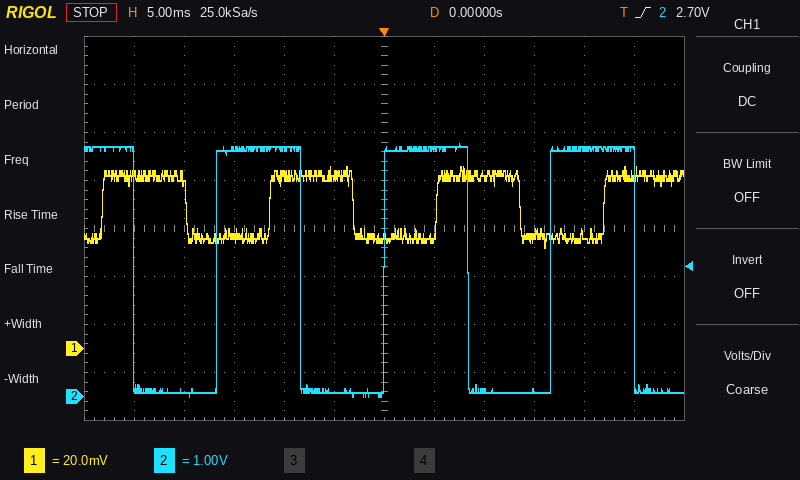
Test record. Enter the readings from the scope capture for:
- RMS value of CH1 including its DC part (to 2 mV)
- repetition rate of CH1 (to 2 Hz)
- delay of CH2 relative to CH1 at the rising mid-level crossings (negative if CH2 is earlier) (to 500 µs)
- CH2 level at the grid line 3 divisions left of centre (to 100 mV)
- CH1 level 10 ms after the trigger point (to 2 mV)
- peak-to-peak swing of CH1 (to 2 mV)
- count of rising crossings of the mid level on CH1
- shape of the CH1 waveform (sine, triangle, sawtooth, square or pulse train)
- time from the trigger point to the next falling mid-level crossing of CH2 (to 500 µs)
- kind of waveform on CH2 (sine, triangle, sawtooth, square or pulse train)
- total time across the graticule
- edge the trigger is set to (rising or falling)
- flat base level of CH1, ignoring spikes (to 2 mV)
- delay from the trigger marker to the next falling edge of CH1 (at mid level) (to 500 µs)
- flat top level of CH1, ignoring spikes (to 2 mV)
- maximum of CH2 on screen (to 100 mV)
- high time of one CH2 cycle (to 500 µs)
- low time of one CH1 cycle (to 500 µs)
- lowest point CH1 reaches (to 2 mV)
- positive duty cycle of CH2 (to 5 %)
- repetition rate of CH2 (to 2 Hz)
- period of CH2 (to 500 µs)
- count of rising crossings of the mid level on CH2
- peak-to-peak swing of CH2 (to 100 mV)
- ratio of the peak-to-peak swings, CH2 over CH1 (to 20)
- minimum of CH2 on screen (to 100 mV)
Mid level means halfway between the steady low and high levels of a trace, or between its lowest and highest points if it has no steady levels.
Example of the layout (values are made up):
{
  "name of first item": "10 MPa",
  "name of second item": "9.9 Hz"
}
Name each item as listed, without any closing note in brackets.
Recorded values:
{
  "RMS value of CH1 including its DC part": "60 mV",
  "repetition rate of CH1": "60 Hz",
  "delay of CH2 relative to CH1 at the rising mid-level crossings (negative if CH2 is earlier)": "-5.5 ms",
  "CH2 level at the grid line 3 divisions left of centre": "5.2 V",
  "CH1 level 10 ms after the trigger point": "72 mV",
  "peak-to-peak swing of CH1": "34 mV",
  "count of rising crossings of the mid level on CH1": "4",
  "shape of the CH1 waveform": "square",
  "time from the trigger point to the next falling mid-level crossing of CH2": "8.5 ms",
  "kind of waveform on CH2": "square",
  "total time across the graticule": "60 ms",
  "edge the trigger is set to": "rising",
  "flat base level of CH1, ignoring spikes": "46 mV",
  "delay from the trigger marker to the next falling edge of CH1 (at mid level)": "13.5 ms",
  "flat top level of CH1, ignoring spikes": "72 mV",
  "maximum of CH2 on screen": "5.3 V",
  "high time of one CH2 cycle": "8.5 ms",
  "low time of one CH1 cycle": "8.5 ms",
  "lowest point CH1 reaches": "42 mV",
  "positive duty cycle of CH2": "50 %",
  "repetition rate of CH2": "60 Hz",
  "period of CH2": "16.5 ms",
  "count of rising crossings of the mid level on CH2": "3",
  "peak-to-peak swing of CH2": "5.3 V",
  "ratio of the peak-to-peak swings, CH2 over CH1": "160",
  "minimum of CH2 on screen": "0.0 V"
}
